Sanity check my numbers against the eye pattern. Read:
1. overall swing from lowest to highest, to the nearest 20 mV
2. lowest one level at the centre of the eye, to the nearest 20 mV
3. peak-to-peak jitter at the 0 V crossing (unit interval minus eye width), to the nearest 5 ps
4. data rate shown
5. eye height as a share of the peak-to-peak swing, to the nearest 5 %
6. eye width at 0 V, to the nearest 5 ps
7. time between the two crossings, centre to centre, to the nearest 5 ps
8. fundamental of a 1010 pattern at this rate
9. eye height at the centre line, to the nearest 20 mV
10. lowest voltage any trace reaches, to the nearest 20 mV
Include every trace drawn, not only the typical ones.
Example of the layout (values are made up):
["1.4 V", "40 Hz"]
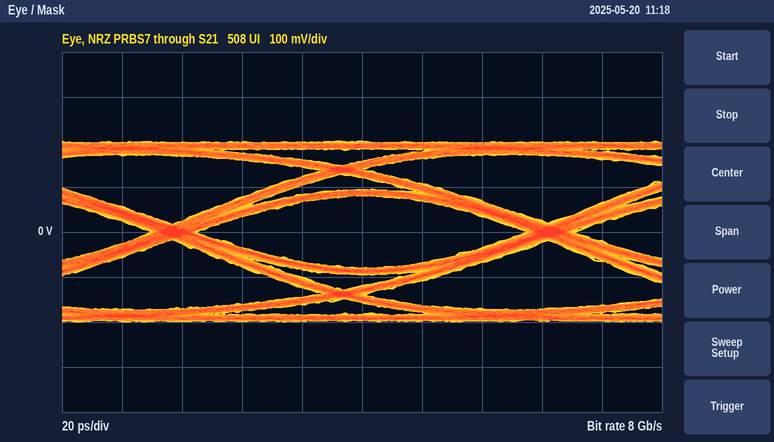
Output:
["400 mV", "80 mV", "15 ps", "8 Gb/s", "40 %", "110 ps", "125 ps", "4 GHz", "160 mV", "-200 mV"]
